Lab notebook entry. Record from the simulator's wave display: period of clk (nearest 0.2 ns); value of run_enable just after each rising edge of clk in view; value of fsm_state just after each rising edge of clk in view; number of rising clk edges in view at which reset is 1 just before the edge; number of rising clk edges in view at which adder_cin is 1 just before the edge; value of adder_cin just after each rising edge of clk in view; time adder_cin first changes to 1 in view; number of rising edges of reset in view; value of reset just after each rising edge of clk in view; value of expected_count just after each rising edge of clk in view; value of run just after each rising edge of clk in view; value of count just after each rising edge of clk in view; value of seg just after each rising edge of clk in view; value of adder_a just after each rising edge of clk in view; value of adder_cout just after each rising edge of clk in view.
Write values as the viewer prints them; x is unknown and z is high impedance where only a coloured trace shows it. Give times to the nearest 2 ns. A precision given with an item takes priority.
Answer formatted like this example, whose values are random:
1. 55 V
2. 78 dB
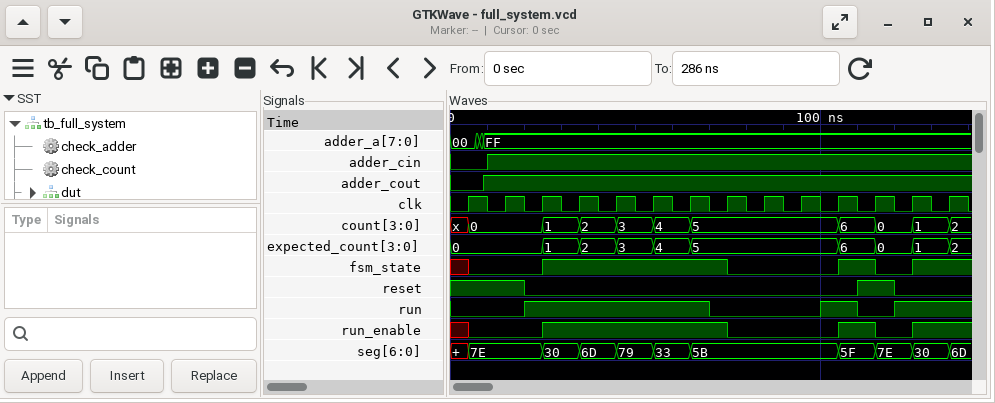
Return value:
1. 10 ns
2. 0 0 1 1 1 1 1 0 0 0 1 0 1 1
3. 0 0 1 1 1 1 1 0 0 0 1 0 1 1
4. 3
5. 13
6. 0 1 1 1 1 1 1 1 1 1 1 1 1 1
7. 10 ns
8. 1
9. 1 1 0 0 0 0 0 0 0 0 0 1 0 0
10. 0, 0, 1, 2, 3, 4, 5, 5, 5, 5, 6, 0, 1, 2
11. 0 0 1 1 1 1 1 0 0 0 1 0 1 1
12. 0, 0, 1, 2, 3, 4, 5, 5, 5, 5, 6, 0, 1, 2
13. 7E, 7E, 30, 6D, 79, 33, 5B, 5B, 5B, 5B, 5F, 7E, 30, 6D
14. 00, FF, FF, FF, FF, FF, FF, FF, FF, FF, FF, FF, FF, FF
15. 0 1 1 1 1 1 1 1 1 1 1 1 1 1
